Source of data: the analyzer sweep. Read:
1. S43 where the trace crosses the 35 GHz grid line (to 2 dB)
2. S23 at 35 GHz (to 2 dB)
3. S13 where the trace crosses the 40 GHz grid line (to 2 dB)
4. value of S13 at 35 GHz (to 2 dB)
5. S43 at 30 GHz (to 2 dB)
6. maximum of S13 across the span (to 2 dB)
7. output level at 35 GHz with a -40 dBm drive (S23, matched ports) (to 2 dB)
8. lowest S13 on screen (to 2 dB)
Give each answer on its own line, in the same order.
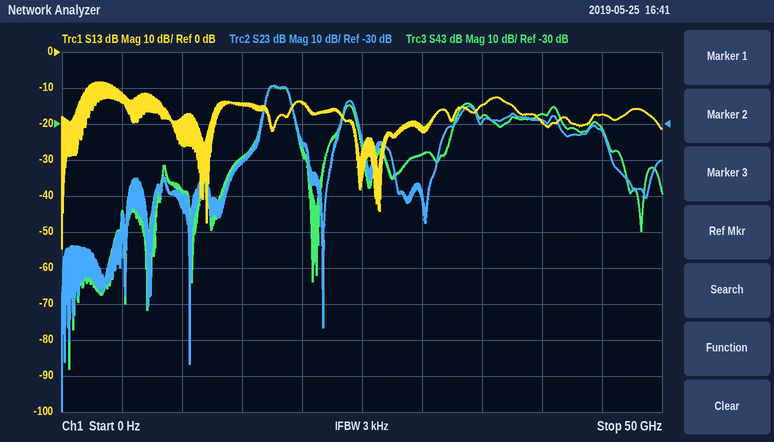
-28 dB
-30 dB
-20 dB
-14 dB
-38 dB
-8 dB
-70 dBm
-54 dB
